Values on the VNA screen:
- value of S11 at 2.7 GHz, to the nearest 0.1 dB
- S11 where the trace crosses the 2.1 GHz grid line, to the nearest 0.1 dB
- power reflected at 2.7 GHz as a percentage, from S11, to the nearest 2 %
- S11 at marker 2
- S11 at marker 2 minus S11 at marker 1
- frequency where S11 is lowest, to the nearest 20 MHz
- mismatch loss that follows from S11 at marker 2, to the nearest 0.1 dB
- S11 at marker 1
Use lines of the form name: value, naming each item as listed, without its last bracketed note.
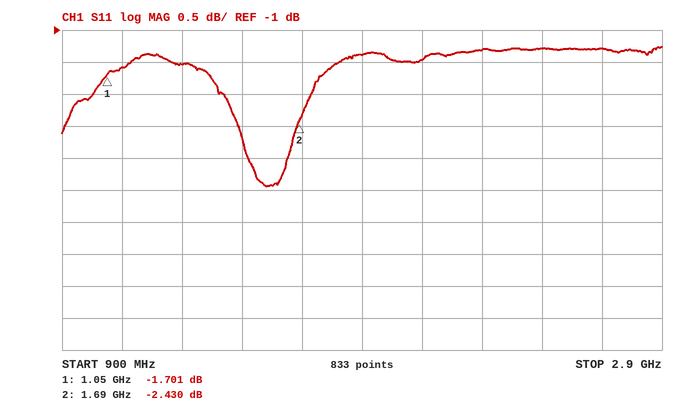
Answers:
value of S11 at 2.7 GHz, to the nearest 0.1 dB: -1.3 dB
S11 where the trace crosses the 2.1 GHz grid line, to the nearest 0.1 dB: -1.5 dB
power reflected at 2.7 GHz as a percentage, from S11, to the nearest 2 %: 74 %
S11 at marker 2: -2.430 dB
S11 at marker 2 minus S11 at marker 1: -0.729 dB
frequency where S11 is lowest, to the nearest 20 MHz: 1.58 GHz
mismatch loss that follows from S11 at marker 2, to the nearest 0.1 dB: 3.7 dB
S11 at marker 1: -1.701 dB
